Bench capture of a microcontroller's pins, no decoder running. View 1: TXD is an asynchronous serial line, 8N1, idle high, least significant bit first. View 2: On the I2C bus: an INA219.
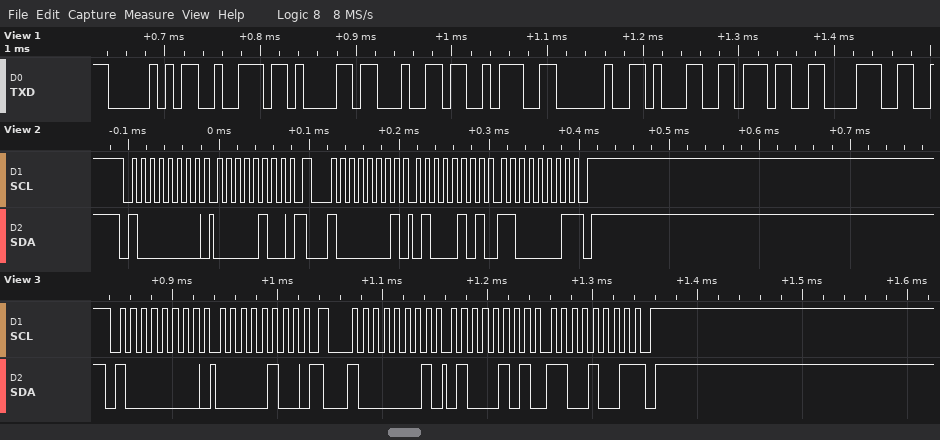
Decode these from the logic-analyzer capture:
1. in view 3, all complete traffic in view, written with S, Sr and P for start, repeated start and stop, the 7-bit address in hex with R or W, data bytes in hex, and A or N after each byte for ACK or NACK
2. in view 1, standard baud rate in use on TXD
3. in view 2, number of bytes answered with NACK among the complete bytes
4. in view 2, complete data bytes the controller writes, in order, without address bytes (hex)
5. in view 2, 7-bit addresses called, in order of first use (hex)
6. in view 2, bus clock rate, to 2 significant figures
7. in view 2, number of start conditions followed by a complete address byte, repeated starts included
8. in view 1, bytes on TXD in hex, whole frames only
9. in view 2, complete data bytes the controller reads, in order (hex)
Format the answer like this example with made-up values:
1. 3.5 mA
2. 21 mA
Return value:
1. S 40W A 04 A Sr 40R A 45 A C9 N P
2. 115200 baud
3. 1
4. 04
5. 0x40
6. 100 kHz
7. 2
8. 0x50 0x72 0x61 0x64 0x3A 0x20 0x31 0x37 0x38
9. 45 C1
